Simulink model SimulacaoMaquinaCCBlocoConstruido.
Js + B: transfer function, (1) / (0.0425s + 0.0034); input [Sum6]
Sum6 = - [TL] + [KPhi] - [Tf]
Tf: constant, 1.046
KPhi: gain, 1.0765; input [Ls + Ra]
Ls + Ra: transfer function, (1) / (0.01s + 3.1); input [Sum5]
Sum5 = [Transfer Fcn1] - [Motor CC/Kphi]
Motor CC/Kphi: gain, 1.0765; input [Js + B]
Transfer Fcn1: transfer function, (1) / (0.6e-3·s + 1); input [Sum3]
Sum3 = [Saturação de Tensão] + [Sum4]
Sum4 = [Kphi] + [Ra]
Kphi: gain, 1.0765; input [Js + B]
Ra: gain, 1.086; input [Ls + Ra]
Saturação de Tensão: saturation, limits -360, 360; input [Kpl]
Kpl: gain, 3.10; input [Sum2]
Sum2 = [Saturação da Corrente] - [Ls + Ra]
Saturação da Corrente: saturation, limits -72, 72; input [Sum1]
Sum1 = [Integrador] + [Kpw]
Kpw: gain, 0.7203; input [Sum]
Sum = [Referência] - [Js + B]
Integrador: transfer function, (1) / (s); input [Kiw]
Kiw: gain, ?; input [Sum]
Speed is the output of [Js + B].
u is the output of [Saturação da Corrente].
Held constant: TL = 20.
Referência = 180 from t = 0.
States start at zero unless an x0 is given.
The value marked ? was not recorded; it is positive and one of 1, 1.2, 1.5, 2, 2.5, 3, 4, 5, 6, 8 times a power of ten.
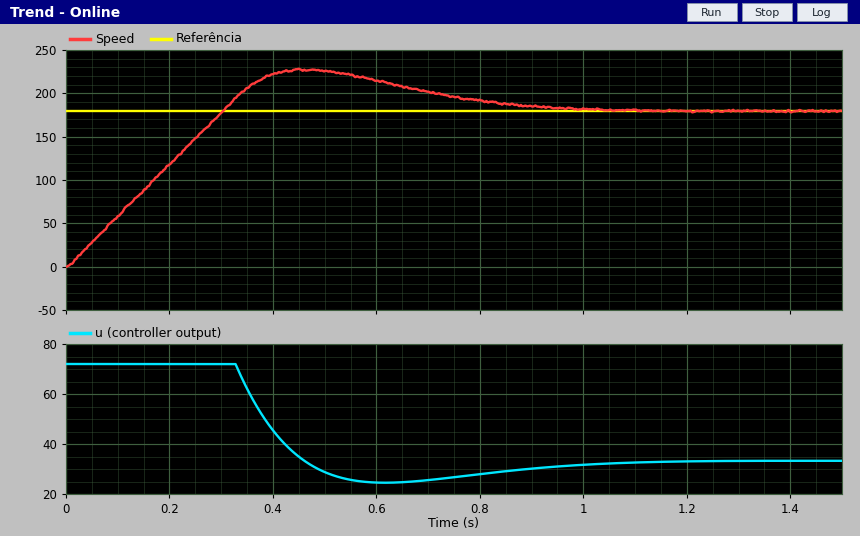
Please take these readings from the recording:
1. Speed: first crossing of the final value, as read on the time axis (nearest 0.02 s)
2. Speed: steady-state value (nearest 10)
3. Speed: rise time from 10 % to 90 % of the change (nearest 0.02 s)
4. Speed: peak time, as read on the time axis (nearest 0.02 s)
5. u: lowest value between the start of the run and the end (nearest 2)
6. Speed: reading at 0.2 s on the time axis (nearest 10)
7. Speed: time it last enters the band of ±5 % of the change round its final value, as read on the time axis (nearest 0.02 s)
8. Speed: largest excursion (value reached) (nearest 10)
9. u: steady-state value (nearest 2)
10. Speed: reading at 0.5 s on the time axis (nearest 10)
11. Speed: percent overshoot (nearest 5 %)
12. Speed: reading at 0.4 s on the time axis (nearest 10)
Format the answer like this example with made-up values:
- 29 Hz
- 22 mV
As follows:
- 0.30 s
- 180
- 0.24 s
- 0.46 s
- 24
- 120
- 0.84 s
- 230
- 34
- 230
- 25 %
- 220
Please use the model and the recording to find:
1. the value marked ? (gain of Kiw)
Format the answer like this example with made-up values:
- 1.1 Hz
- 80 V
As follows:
- 3
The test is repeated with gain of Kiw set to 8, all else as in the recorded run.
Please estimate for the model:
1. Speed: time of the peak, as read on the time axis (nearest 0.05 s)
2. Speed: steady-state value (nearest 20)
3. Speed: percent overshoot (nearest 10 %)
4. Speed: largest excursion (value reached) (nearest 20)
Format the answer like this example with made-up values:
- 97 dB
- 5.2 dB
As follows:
- 0.50 s
- 180
- 60 %
- 300
